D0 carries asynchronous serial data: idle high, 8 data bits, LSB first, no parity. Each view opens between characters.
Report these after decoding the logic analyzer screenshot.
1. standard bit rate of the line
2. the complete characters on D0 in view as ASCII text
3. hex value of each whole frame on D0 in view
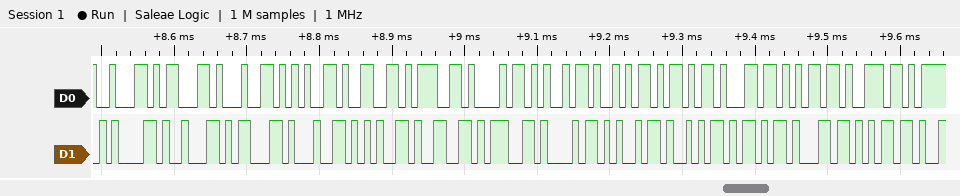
115200 baud
"bcdefghijklmn"
62, 63, 64, 65, 66, 67, 68, 69, 6A, 6B, 6C, 6D, 6E
